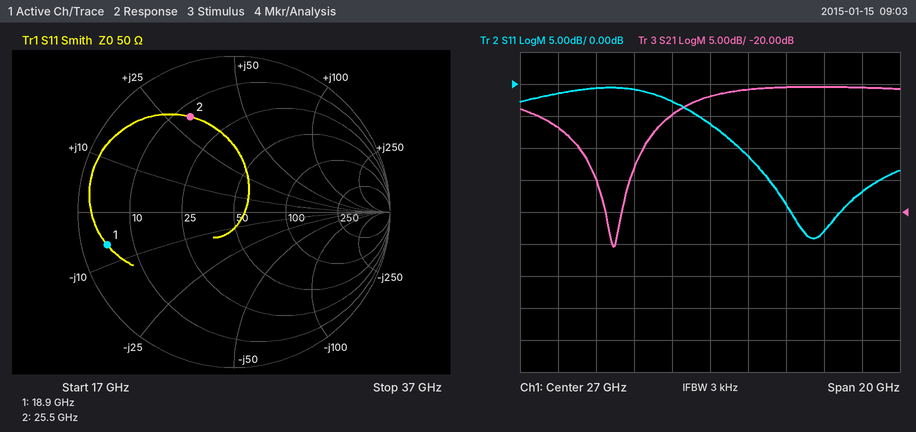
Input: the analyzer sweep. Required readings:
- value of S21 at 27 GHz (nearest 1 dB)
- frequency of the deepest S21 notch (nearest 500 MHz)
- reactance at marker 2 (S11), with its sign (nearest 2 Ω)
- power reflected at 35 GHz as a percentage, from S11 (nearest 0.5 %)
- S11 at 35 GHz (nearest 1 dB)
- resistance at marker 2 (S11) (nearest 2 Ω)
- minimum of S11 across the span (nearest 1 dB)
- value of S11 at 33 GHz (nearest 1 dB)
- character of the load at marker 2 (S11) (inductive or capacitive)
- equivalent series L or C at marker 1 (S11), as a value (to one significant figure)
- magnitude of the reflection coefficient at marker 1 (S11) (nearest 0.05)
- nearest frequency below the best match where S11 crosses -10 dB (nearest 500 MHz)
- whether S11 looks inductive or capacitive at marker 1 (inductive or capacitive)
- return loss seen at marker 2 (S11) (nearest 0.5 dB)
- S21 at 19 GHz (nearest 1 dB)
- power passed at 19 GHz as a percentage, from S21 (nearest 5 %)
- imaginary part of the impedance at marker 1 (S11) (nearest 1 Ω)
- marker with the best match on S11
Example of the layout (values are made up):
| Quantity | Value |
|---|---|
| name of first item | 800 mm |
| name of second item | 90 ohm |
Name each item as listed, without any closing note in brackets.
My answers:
| Quantity | Value |
|---|---|
| value of S21 at 27 GHz | -2 dB |
| frequency of the deepest S21 notch | 22.0 GHz |
| reactance at marker 2 (S11), with its sign | +30 Ω |
| power reflected at 35 GHz as a percentage, from S11 | 2.0 % |
| S11 at 35 GHz | -17 dB |
| resistance at marker 2 (S11) | 14 Ω |
| minimum of S11 across the span | -24 dB |
| value of S11 at 33 GHz | -23 dB |
| character of the load at marker 2 (S11) | inductive |
| equivalent series L or C at marker 1 (S11), as a value | 1 pF |
| magnitude of the reflection coefficient at marker 1 (S11) | 0.85 |
| nearest frequency below the best match where S11 crosses -10 dB | 28.5 GHz |
| whether S11 looks inductive or capacitive at marker 1 | capacitive |
| return loss seen at marker 2 (S11) | 3.5 dB |
| S21 at 19 GHz | -7 dB |
| power passed at 19 GHz as a percentage, from S21 | 20 % |
| imaginary part of the impedance at marker 1 (S11) | -6 Ω |
| marker with the best match on S11 | marker 2 |
